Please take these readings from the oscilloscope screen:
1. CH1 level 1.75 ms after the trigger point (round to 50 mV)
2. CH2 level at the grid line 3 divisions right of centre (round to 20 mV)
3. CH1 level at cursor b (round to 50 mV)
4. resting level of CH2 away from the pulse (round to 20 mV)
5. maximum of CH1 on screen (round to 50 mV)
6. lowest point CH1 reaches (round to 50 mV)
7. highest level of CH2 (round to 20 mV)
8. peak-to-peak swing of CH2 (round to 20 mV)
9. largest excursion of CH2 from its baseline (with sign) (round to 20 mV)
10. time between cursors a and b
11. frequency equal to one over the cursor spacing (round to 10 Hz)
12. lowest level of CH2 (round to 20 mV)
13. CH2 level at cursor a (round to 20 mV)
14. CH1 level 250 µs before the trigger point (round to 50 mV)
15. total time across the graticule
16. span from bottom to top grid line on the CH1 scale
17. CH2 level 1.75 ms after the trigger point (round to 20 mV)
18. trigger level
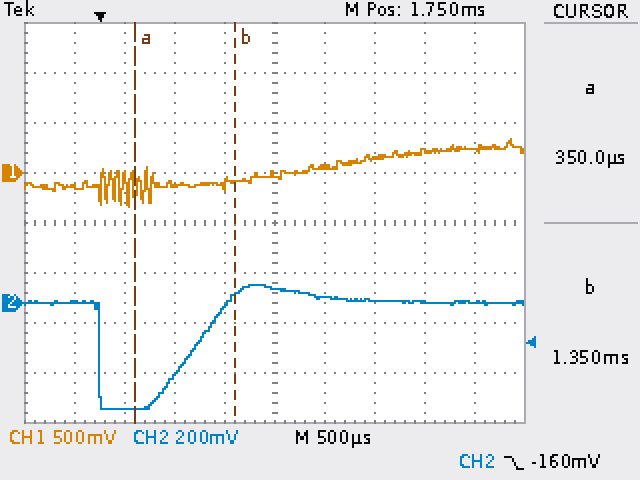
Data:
0 mV
0 mV
-100 mV
0 mV
350 mV
-350 mV
80 mV
500 mV
-420 mV
1.00 ms
1.00 kHz
-420 mV
-420 mV
-150 mV
5 ms
4 V
60 mV
-160 mV
